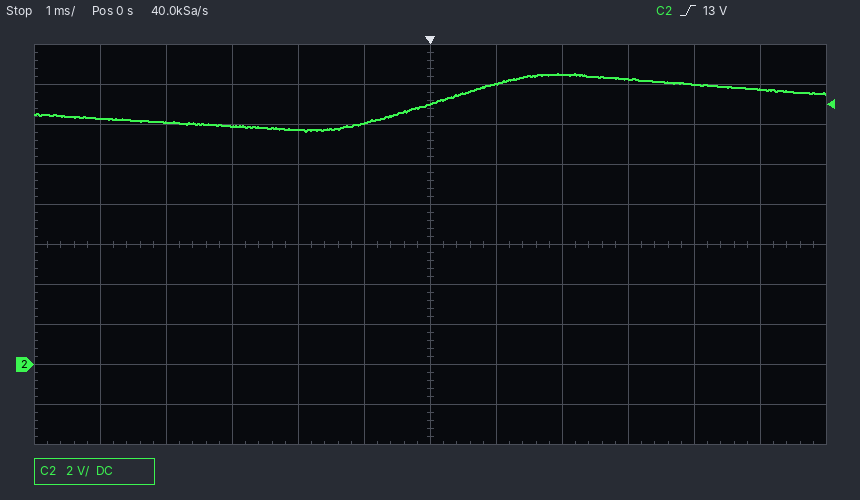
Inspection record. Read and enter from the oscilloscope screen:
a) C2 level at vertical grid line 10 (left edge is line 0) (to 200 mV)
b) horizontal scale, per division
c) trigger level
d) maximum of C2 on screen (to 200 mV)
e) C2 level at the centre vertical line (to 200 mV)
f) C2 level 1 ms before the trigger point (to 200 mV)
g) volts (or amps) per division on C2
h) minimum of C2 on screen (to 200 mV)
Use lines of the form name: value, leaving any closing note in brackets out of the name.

C2 level at vertical grid line 10 (left edge is line 0): 14.0 V
horizontal scale, per division: 1 ms
trigger level: 13 V
maximum of C2 on screen: 14.6 V
C2 level at the centre vertical line: 13.0 V
C2 level 1 ms before the trigger point: 12.0 V
volts (or amps) per division on C2: 2 V
minimum of C2 on screen: 11.6 V
